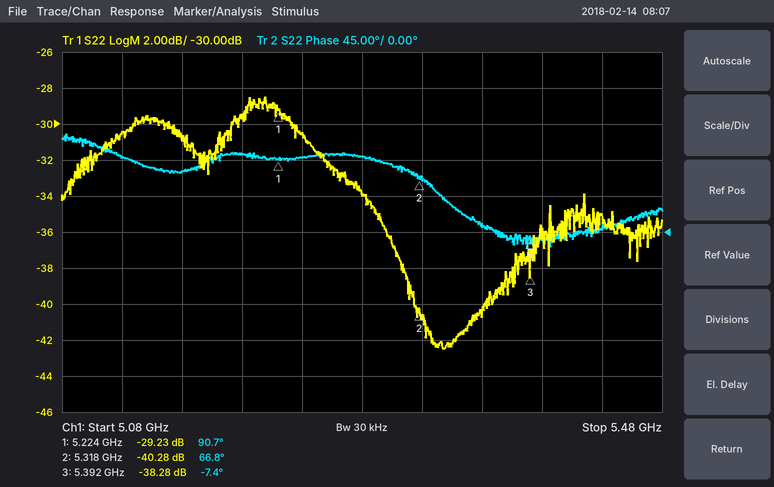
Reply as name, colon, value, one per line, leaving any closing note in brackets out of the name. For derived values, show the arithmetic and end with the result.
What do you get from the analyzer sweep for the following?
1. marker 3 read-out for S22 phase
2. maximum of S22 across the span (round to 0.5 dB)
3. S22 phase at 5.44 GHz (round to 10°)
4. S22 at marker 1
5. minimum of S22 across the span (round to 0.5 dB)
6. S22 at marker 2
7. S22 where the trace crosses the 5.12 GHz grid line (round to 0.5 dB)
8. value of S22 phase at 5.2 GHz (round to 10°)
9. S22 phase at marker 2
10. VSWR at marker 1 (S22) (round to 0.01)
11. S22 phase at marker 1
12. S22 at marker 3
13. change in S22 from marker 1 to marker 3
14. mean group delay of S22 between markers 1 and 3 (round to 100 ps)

marker 3 read-out for S22 phase: -7.4°
maximum of S22 across the span: -28.5 dB
S22 phase at 5.44 GHz: 0°
S22 at marker 1: -29.23 dB
minimum of S22 across the span: -42.5 dB
S22 at marker 2: -40.28 dB
S22 where the trace crosses the 5.12 GHz grid line: -30.5 dB
value of S22 phase at 5.2 GHz: 100°
S22 phase at marker 2: 66.8°
VSWR at marker 1 (S22): (1 + 0.0346)/(1 − 0.0346) ≈ 1.07
S22 phase at marker 1: 90.7°
S22 at marker 3: -38.28 dB
change in S22 from marker 1 to marker 3: -38.28 − (-29.23) = -9.05 dB
mean group delay of S22 between markers 1 and 3: −(-7.4° − (90.7°))/(360° × 168 MHz) ≈ 1.6 ns
